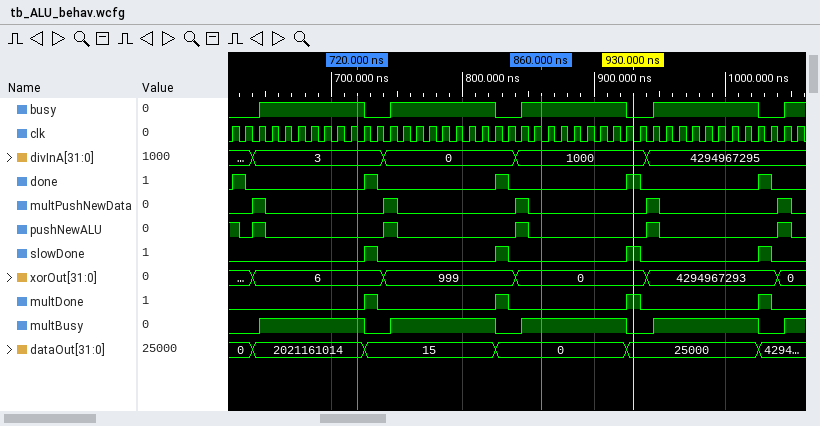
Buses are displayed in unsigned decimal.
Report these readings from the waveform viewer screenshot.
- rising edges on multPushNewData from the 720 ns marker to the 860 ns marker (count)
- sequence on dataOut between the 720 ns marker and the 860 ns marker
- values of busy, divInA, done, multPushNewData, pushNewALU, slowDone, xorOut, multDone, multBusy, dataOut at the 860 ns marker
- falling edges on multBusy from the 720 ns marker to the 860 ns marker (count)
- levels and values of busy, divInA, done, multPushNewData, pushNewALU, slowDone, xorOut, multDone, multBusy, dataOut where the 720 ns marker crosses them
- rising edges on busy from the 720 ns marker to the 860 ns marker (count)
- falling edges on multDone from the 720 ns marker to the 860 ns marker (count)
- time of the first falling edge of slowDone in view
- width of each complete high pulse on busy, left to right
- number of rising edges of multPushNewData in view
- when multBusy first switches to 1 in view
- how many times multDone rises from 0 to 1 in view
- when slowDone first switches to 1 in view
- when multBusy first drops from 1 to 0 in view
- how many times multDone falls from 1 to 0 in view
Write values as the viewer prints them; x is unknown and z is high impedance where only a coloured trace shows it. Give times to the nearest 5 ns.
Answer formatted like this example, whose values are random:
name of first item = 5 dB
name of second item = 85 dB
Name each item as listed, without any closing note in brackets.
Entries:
rising edges on multPushNewData from the 720 ns marker to the 860 ns marker = 2
sequence on dataOut between the 720 ns marker and the 860 ns marker = 2021161014, 15, 0
values of busy, divInA, done, multPushNewData, pushNewALU, slowDone, xorOut, multDone, multBusy, dataOut at the 860 ns marker = busy=1, divInA=1000, done=0, multPushNewData=0, pushNewALU=0, slowDone=0, xorOut=0, multDone=0, multBusy=1, dataOut=0
falling edges on multBusy from the 720 ns marker to the 860 ns marker = 2
levels and values of busy, divInA, done, multPushNewData, pushNewALU, slowDone, xorOut, multDone, multBusy, dataOut where the 720 ns marker crosses them = busy=1, divInA=3, done=0, multPushNewData=0, pushNewALU=0, slowDone=0, xorOut=6, multDone=0, multBusy=1, dataOut=2021161014
rising edges on busy from the 720 ns marker to the 860 ns marker = 2
falling edges on multDone from the 720 ns marker to the 860 ns marker = 2
time of the first falling edge of slowDone in view = 735 ns
width of each complete high pulse on busy, left to right = 80 ns, 80 ns, 80 ns, 80 ns
number of rising edges of multPushNewData in view = 5
when multBusy first switches to 1 in view = 645 ns
how many times multDone rises from 0 to 1 in view = 4
when slowDone first switches to 1 in view = 725 ns
when multBusy first drops from 1 to 0 in view = 725 ns
how many times multDone falls from 1 to 0 in view = 4
